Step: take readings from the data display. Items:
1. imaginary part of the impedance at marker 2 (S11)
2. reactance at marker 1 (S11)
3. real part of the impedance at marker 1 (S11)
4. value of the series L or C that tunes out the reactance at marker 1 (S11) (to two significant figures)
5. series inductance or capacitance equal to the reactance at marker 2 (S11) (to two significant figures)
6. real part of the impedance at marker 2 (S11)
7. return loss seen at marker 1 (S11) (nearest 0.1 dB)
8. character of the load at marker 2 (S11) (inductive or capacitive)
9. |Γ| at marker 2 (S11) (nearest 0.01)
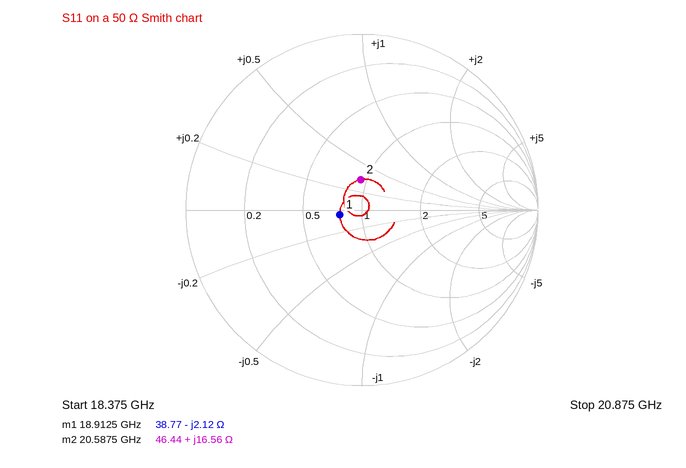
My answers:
+16.56 Ω
-2.12 Ω
38.77 Ω
18 pH
130 pH
46.44 Ω
17.8 dB
inductive
0.17
